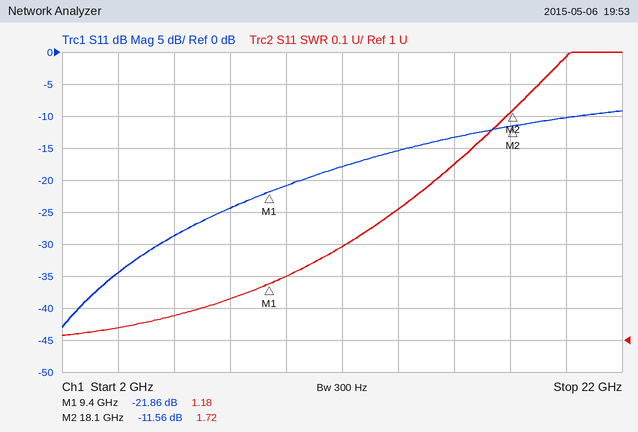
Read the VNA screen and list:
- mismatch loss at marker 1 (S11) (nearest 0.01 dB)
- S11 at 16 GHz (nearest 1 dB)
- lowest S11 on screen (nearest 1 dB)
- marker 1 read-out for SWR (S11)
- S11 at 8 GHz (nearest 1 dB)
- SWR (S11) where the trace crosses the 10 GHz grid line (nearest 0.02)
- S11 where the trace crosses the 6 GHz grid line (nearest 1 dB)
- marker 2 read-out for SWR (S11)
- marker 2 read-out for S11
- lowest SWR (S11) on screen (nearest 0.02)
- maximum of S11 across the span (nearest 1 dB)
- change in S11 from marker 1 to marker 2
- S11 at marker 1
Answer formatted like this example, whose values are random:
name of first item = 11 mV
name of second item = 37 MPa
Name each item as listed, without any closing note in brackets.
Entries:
mismatch loss at marker 1 (S11) = 0.03 dB
S11 at 16 GHz = -13 dB
lowest S11 on screen = -43 dB
marker 1 read-out for SWR = 1.18
S11 at 8 GHz = -24 dB
SWR (S11) where the trace crosses the 10 GHz grid line = 1.20
S11 where the trace crosses the 6 GHz grid line = -29 dB
marker 2 read-out for SWR = 1.72
marker 2 read-out for S11 = -11.56 dB
lowest SWR (S11) on screen = 1.02
maximum of S11 across the span = -9 dB
change in S11 from marker 1 to marker 2 = 10.30 dB
S11 at marker 1 = -21.86 dB
